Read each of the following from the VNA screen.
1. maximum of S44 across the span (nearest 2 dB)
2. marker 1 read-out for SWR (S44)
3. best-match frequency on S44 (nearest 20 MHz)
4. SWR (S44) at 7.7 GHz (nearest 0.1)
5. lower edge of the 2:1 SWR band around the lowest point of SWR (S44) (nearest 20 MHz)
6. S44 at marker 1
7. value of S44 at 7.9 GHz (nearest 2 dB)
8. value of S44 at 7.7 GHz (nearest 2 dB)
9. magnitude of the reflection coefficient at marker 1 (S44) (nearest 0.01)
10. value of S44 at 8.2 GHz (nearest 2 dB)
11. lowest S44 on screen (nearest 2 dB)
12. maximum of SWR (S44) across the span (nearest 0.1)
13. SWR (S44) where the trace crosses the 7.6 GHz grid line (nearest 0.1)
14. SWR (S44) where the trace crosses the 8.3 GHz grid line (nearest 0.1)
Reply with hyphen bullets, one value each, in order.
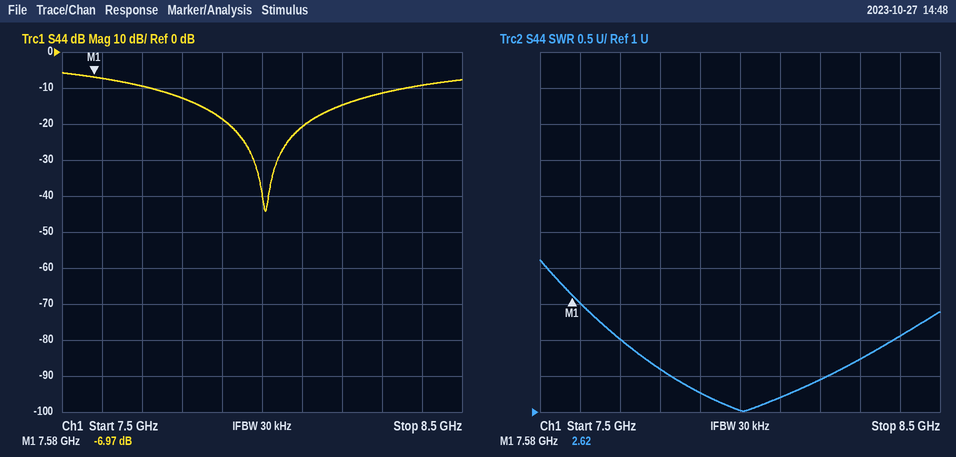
- -6 dB
- 2.62
- 8.00 GHz
- 2.0
- 7.70 GHz
- -6.97 dB
- -18 dB
- -10 dB
- 0.45
- -14 dB
- -44 dB
- 3.1
- 2.5
- 1.7
